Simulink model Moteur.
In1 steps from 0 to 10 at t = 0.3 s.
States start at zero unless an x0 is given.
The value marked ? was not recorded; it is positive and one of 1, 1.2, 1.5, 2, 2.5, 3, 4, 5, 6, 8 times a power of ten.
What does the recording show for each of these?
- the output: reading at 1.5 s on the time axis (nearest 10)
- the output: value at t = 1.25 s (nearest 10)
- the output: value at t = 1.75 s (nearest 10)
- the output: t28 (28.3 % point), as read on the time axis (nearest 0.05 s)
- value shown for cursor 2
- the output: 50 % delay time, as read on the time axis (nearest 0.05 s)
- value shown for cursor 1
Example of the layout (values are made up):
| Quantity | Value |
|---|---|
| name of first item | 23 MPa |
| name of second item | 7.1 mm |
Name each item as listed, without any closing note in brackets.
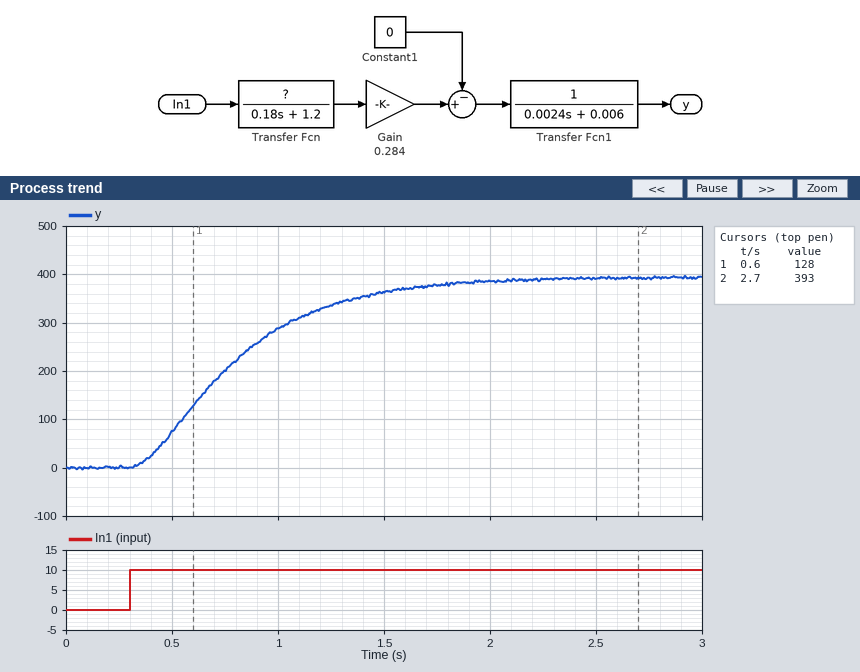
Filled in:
| Quantity | Value |
|---|---|
| the output: reading at 1.5 s on the time axis | 360 |
| the output: value at t = 1.25 s | 340 |
| the output: value at t = 1.75 s | 380 |
| the output: t28 (28.3 % point), as read on the time axis | 0.55 s |
| value shown for cursor 2 | 393 |
| the output: 50 % delay time, as read on the time axis | 0.75 s |
| value shown for cursor 1 | 128 |
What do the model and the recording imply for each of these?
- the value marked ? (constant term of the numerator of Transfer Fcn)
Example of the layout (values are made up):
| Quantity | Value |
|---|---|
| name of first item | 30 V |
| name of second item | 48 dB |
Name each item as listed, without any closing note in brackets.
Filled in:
| Quantity | Value |
|---|---|
| the value marked ? | 1 |
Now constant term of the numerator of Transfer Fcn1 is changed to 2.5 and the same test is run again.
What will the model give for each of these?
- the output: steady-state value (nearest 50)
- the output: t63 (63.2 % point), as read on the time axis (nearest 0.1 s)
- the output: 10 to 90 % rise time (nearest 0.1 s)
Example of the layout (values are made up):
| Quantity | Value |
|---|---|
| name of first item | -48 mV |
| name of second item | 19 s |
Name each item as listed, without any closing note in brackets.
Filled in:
| Quantity | Value |
|---|---|
| the output: steady-state value | 1000 |
| the output: t63 (63.2 % point), as read on the time axis | 0.9 s |
| the output: 10 to 90 % rise time | 1.0 s |
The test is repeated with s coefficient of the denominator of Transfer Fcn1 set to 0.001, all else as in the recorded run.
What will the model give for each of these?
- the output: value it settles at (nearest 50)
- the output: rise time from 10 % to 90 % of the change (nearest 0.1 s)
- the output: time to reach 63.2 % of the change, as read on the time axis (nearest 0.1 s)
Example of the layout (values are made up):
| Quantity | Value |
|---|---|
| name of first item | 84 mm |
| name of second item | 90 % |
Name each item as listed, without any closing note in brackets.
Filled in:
| Quantity | Value |
|---|---|
| the output: value it settles at | 400 |
| the output: rise time from 10 % to 90 % of the change | 0.5 s |
| the output: time to reach 63.2 % of the change, as read on the time axis | 0.6 s |
